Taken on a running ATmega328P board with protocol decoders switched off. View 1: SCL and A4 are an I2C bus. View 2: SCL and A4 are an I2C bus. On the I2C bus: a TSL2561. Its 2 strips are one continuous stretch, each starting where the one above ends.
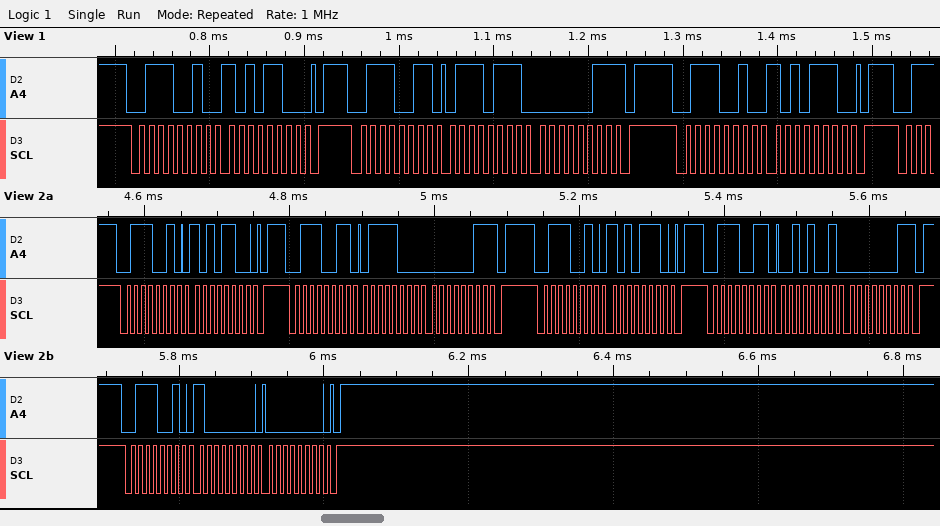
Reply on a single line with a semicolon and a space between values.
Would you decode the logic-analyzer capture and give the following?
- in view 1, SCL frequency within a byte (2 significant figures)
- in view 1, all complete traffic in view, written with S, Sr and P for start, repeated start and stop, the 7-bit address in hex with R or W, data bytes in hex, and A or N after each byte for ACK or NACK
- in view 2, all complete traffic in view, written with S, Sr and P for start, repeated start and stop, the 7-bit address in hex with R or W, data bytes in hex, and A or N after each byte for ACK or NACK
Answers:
100 kHz; S 39W A AC A P S 39R A 77 A 03 N P S 39W A AE A P; S 39W A AC A P S 39R A 78 A 03 N P S 39W A AE A P S 39R A 29 A 01 N P S 39W A 80 A 00 A P
